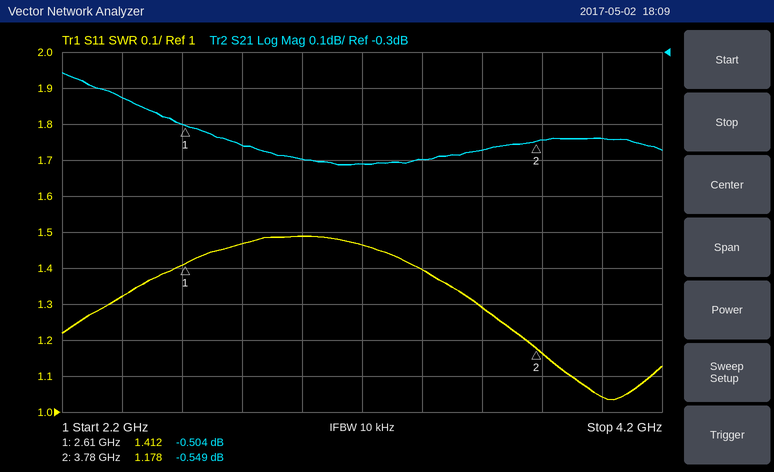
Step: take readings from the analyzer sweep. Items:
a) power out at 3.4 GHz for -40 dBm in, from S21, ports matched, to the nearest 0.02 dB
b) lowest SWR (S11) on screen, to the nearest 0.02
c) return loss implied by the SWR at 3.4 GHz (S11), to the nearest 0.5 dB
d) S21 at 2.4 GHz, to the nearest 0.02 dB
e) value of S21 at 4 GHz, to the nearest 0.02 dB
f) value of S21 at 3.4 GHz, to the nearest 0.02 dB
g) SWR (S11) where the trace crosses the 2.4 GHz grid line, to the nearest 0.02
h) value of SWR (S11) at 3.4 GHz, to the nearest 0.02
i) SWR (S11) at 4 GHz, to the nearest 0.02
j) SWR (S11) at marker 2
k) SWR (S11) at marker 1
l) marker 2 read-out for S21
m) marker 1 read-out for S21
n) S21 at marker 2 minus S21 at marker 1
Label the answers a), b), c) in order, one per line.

a) -40.60 dBm
b) 1.04
c) 15.5 dB
d) -0.42 dB
e) -0.54 dB
f) -0.60 dB
g) 1.32
h) 1.40
i) 1.04
j) 1.178
k) 1.412
l) -0.549 dB
m) -0.504 dB
n) -0.045 dB
